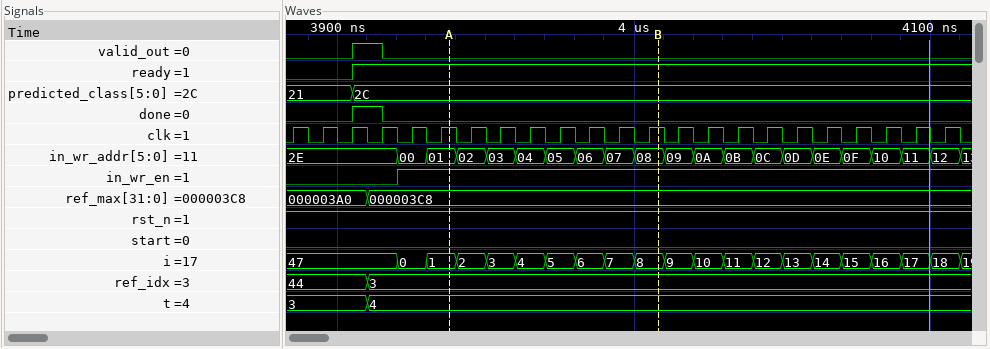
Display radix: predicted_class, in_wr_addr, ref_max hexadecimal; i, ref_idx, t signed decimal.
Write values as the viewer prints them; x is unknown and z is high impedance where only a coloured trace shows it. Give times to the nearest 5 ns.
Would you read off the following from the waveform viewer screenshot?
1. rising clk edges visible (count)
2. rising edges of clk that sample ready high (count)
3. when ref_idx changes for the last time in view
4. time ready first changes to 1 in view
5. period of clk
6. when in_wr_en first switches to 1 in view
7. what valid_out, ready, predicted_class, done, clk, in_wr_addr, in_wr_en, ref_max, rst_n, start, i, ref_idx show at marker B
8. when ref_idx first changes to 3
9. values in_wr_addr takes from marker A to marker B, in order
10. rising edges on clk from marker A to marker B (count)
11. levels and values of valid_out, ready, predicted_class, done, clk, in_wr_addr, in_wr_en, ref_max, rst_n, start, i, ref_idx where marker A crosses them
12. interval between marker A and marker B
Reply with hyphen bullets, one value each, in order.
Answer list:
- 23
- 20
- 3910 ns
- 3905 ns
- 10 ns
- 3920 ns
- valid_out=0, ready=1, predicted_class=2C, done=0, clk=1, in_wr_addr=08, in_wr_en=1, ref_max=000003C8, rst_n=1, start=0, i=8, ref_idx=3
- 3910 ns
- 01, 02, 03, 04, 05, 06, 07, 08
- 7
- valid_out=0, ready=1, predicted_class=2C, done=0, clk=1, in_wr_addr=01, in_wr_en=1, ref_max=000003C8, rst_n=1, start=0, i=1, ref_idx=3
- 70 ns
